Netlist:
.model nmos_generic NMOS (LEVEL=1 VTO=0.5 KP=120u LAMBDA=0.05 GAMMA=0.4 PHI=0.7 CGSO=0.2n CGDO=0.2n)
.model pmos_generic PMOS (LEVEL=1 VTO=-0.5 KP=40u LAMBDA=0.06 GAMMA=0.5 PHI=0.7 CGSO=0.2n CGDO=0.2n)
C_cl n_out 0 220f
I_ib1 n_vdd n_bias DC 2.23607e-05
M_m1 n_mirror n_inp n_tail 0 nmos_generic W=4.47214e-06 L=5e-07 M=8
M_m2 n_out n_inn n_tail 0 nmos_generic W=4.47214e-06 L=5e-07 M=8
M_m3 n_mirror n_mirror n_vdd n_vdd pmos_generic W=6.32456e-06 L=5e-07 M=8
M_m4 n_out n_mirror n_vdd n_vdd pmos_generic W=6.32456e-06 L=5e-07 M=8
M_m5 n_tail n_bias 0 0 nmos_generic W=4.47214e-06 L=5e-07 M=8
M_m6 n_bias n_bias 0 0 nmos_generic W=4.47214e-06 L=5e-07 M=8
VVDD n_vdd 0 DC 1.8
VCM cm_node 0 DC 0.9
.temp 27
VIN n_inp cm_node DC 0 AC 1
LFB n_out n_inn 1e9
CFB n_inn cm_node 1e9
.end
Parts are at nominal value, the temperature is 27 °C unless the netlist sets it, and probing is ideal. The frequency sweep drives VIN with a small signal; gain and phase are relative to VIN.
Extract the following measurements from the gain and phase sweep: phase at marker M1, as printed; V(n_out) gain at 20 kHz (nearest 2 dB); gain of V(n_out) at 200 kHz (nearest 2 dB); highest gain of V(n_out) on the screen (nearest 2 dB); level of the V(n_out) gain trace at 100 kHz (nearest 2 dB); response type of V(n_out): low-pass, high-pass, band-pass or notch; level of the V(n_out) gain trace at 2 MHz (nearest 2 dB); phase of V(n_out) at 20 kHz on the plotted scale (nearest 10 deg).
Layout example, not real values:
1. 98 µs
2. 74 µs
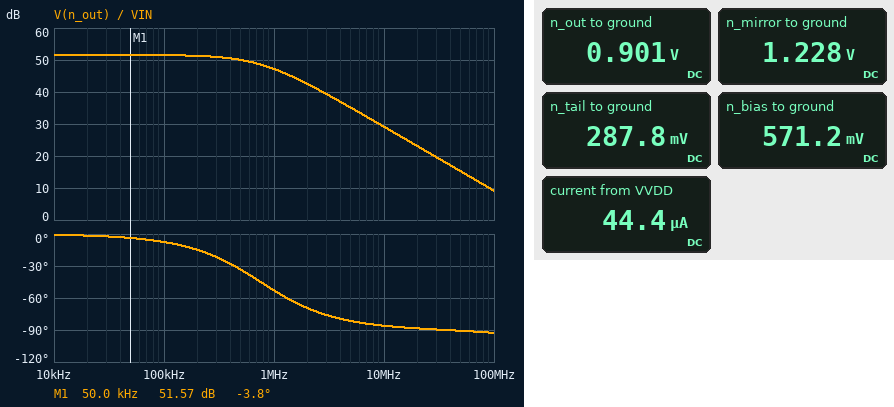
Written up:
1. -3.8 deg
2. 52 dB
3. 52 dB
4. 52 dB
5. 52 dB
6. low-pass
7. 42 dB
8. 0 deg
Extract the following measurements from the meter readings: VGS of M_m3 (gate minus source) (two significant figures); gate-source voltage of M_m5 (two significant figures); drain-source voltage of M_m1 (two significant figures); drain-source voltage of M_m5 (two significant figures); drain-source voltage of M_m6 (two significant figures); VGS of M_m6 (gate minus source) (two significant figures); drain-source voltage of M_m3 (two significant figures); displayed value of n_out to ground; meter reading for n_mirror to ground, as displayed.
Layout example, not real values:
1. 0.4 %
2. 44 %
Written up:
1. -570 mV
2. 570 mV
3. 940 mV
4. 290 mV
5. 570 mV
6. 570 mV
7. -570 mV
8. 0.901 V
9. 1.228 V
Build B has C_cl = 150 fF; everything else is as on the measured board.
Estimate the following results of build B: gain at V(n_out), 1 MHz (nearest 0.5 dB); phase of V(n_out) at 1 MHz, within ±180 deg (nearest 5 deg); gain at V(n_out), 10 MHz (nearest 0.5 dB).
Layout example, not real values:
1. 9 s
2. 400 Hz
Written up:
1. 49.0 dB
2. -45 deg
3. 32.0 dB
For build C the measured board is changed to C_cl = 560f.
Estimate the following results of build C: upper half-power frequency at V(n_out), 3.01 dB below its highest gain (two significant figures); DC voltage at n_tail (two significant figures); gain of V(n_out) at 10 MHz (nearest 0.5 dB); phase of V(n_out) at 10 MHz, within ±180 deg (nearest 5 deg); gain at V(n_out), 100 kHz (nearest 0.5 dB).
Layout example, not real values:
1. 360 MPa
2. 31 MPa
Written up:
1. 320 kHz
2. 290 mV
3. 21.5 dB
4. -90 deg
5. 51.0 dB
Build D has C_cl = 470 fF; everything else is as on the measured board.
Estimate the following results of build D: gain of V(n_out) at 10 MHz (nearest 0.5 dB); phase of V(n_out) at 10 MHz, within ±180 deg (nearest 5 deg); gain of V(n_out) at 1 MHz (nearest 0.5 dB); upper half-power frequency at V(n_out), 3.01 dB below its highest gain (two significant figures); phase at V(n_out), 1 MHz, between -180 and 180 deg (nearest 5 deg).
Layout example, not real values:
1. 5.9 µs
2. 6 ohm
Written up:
1. 23.0 dB
2. -90 deg
3. 42.5 dB
4. 380 kHz
5. -70 deg
